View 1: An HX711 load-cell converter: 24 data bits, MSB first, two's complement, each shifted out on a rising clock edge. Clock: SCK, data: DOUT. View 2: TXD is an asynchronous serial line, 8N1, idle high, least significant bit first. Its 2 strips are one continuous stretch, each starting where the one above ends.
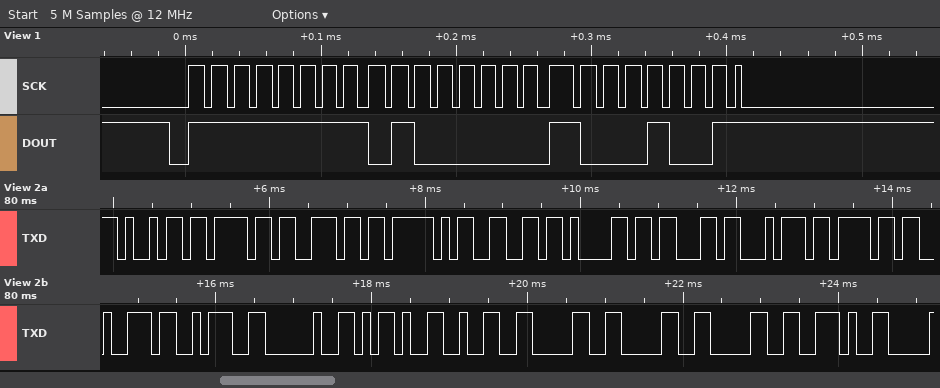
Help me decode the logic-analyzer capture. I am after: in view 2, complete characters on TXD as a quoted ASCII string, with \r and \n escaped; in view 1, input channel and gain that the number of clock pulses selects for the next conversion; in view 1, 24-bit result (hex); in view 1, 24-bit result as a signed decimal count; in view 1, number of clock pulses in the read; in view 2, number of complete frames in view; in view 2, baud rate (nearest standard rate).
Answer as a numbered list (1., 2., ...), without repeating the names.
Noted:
1. "ion_factor: -2000."
2. channel A, gain 128
3. 0xFF4089
4. -49015
5. 25
6. 18
7. 9600 baud
